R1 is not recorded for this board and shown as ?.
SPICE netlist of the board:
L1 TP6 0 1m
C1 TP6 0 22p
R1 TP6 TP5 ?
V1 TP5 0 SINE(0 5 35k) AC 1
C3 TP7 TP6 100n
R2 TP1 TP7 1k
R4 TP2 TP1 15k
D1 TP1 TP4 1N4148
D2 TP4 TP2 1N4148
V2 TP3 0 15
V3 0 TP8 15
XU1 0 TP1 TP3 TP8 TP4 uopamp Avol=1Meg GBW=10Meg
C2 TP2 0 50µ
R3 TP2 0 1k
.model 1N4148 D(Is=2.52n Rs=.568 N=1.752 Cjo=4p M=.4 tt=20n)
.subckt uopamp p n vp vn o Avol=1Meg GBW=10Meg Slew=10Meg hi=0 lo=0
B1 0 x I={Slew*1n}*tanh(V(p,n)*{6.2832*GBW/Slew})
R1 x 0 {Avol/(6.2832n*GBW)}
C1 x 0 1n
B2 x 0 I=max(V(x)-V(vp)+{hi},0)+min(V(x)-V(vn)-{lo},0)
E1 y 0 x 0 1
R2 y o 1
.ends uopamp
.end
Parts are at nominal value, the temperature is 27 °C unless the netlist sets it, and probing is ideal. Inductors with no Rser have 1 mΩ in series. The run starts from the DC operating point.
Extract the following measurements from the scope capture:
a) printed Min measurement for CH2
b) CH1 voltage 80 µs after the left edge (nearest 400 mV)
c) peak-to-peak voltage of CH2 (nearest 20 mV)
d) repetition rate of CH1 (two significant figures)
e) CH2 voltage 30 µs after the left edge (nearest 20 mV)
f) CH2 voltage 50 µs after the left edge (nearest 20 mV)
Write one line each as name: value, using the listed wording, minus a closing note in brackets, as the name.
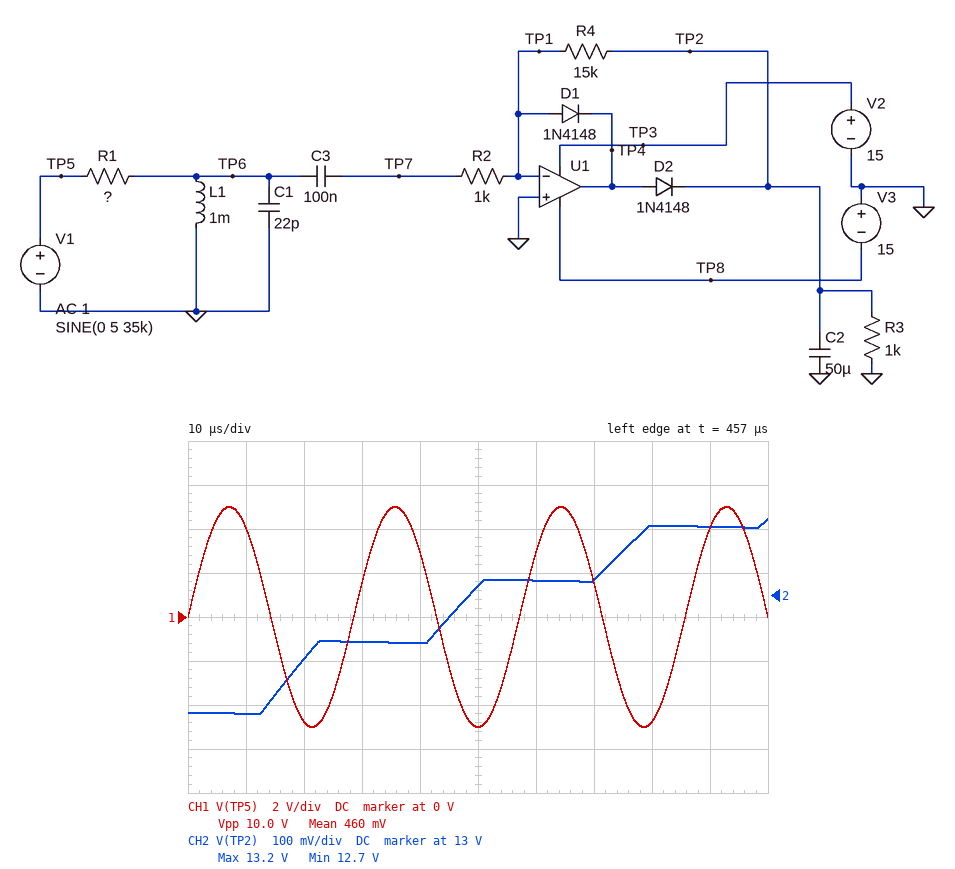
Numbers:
printed Min measurement for CH2: 12.7 V
CH1 voltage 80 µs after the left edge: -4.8 V
peak-to-peak voltage of CH2: 440 mV
repetition rate of CH1: 35 kHz
CH2 voltage 30 µs after the left edge: 12.90 V
CH2 voltage 50 µs after the left edge: 13.02 V
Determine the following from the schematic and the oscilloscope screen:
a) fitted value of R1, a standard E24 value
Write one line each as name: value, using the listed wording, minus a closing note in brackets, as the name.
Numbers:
fitted value of R1, a standard E24 value: 470 Ω
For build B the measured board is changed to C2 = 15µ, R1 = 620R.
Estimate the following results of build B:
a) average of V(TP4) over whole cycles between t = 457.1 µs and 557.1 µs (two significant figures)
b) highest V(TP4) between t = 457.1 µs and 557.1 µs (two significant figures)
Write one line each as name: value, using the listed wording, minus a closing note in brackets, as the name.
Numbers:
average of V(TP4) over whole cycles between t = 457.1 µs and 557.1 µs: 4.3 V
highest V(TP4) between t = 457.1 µs and 557.1 µs: 15 V
